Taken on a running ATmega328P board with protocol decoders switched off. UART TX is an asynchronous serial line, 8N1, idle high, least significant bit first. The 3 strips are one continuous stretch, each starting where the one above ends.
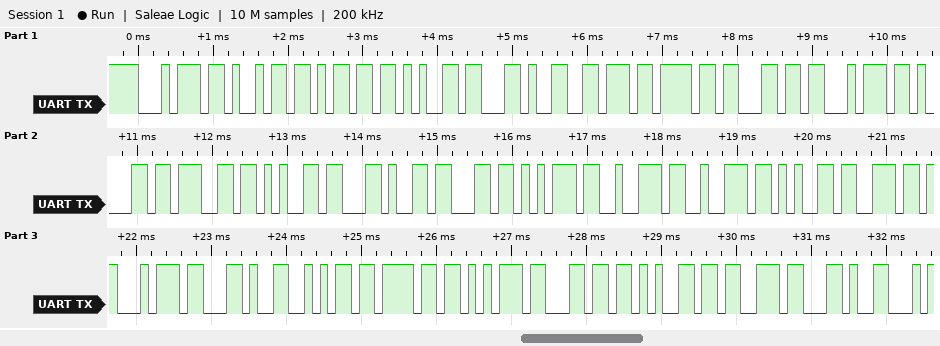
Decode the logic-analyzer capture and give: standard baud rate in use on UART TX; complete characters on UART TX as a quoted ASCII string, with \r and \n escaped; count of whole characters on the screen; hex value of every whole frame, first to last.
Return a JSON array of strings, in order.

["9600 baud", "\"time,voltage,current,joules,\"", "28", "0x74 0x69 0x6D 0x65 0x2C 0x76 0x6F 0x6C 0x74 0x61 0x67 0x65 0x2C 0x63 0x75 0x72 0x72 0x65 0x6E 0x74 0x2C 0x6A 0x6F 0x75 0x6C 0x65 0x73 0x2C"]
